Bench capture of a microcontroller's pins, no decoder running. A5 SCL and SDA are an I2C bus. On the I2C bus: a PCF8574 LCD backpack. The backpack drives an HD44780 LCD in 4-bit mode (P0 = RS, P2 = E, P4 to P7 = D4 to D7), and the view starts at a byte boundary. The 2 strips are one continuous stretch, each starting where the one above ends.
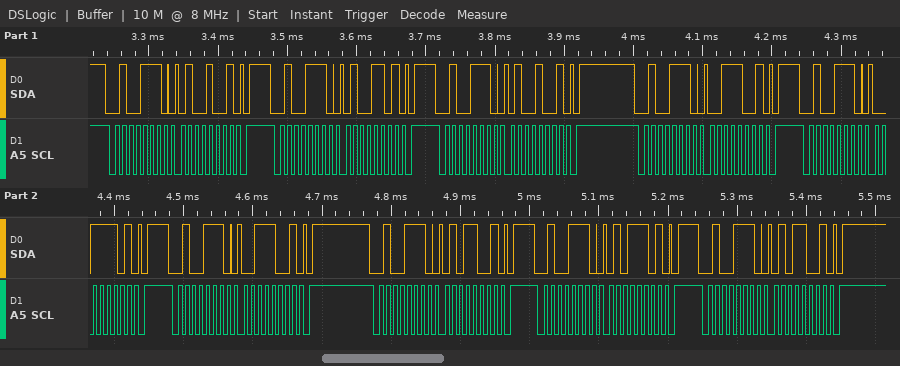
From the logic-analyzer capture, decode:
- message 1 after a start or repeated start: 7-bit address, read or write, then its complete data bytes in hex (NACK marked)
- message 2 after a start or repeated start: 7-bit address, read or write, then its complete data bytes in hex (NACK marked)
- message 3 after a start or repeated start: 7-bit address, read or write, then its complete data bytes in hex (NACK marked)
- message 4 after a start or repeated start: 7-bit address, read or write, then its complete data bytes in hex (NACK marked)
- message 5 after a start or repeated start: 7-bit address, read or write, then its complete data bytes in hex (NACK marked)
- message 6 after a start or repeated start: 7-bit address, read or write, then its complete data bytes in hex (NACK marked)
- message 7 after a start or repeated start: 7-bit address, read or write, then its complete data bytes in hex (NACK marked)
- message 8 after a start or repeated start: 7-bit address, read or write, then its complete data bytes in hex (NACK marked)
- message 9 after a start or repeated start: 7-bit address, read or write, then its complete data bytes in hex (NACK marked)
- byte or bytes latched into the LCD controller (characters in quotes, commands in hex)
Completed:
0x27 write: 49
0x27 write: 4D
0x27 write: 49
0x27 write: 39
0x27 write: 3D
0x27 write: 39
0x27 write: 59
0x27 write: 5D
0x27 write: 59
'C'
